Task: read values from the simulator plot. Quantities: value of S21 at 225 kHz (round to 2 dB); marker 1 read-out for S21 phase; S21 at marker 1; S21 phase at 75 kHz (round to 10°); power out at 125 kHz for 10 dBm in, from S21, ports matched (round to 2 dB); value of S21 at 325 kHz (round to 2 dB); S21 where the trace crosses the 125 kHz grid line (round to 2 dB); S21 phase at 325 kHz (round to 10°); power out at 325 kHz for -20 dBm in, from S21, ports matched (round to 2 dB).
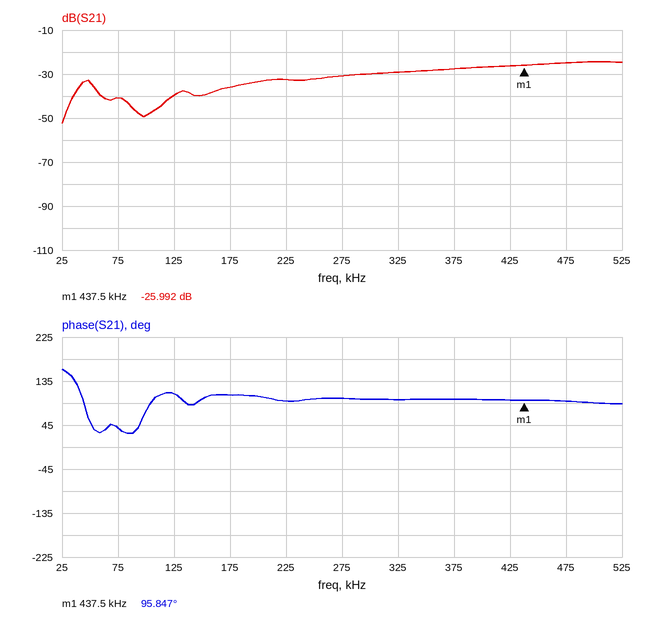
-32 dB
95.847°
-25.992 dB
40°
-30 dBm
-30 dB
-40 dB
100°
-50 dBm
